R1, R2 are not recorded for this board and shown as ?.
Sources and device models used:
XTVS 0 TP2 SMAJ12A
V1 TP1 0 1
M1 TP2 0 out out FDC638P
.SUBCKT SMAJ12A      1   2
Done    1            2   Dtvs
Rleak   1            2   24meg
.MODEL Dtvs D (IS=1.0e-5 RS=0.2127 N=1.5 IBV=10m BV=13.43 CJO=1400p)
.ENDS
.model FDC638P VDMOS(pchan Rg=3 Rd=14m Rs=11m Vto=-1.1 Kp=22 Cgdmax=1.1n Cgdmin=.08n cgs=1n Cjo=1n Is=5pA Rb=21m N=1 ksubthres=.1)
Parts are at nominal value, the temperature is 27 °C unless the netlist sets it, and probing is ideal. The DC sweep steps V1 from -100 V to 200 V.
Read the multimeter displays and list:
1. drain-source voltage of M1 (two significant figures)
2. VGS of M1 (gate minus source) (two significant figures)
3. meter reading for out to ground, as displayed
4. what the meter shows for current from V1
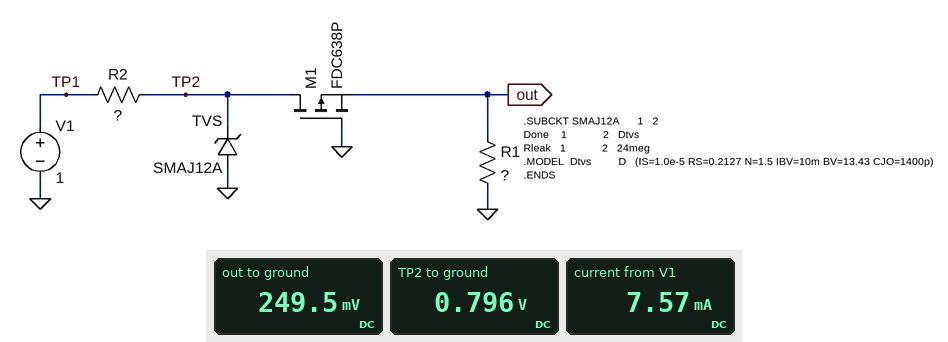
550 mV
-250 mV
249.5 mV
7.57 mA
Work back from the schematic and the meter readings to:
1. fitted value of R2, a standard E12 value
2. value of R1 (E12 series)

27 Ω
33 Ω
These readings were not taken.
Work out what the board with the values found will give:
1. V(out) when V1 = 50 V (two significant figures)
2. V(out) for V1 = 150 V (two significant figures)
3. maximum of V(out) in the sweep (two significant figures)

14 V
15 V
15 V
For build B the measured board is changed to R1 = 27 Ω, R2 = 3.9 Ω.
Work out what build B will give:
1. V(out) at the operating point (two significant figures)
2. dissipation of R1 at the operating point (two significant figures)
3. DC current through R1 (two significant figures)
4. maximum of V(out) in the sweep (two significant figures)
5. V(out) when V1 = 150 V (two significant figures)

390 mV
5.6 mW
14 mA
23 V
21 V
